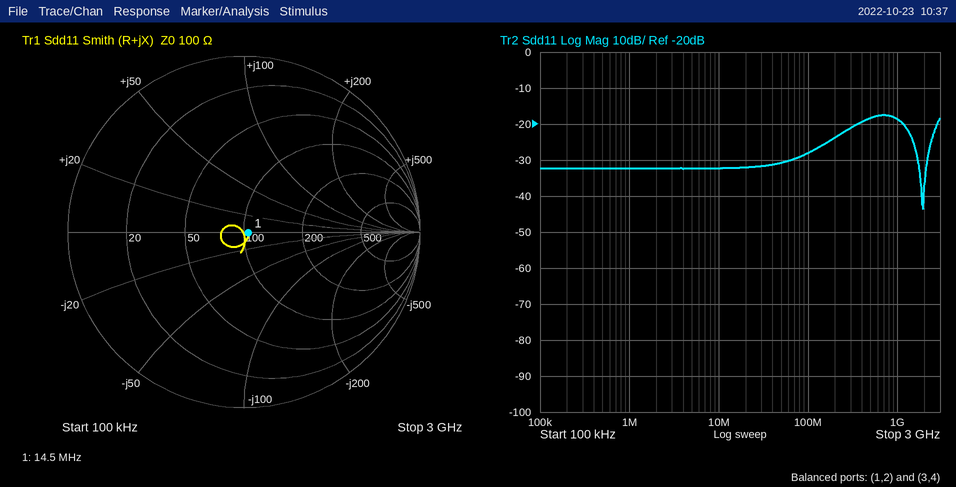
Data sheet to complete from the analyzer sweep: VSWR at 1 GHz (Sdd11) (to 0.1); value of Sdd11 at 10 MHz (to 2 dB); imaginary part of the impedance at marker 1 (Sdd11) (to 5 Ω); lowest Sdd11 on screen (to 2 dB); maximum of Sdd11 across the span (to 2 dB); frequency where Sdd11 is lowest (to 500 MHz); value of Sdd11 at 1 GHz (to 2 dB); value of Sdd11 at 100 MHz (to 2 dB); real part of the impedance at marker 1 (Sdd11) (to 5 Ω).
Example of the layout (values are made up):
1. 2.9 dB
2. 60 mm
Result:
1. 1.3
2. -32 dB
3. 0 Ω
4. -44 dB
5. -18 dB
6. 2.0 GHz
7. -18 dB
8. -28 dB
9. 105 Ω
